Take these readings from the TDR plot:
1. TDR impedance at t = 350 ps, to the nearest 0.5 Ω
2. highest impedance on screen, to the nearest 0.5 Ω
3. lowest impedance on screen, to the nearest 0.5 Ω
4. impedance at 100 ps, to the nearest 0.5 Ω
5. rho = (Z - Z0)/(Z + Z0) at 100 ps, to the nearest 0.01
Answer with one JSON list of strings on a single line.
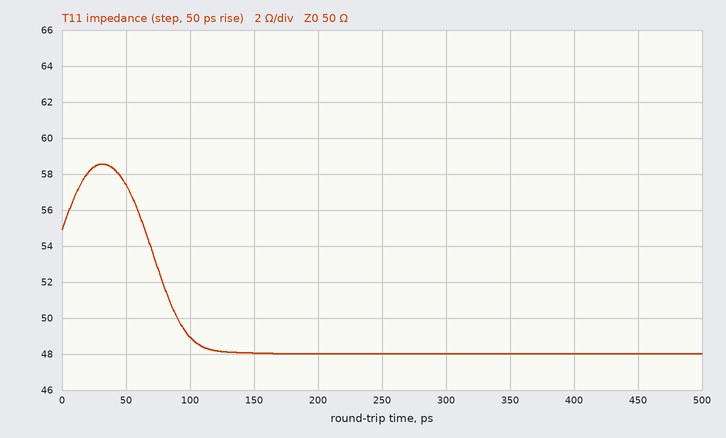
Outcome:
["48.0 Ω", "58.5 Ω", "48.0 Ω", "49.0 Ω", "-0.01"]
